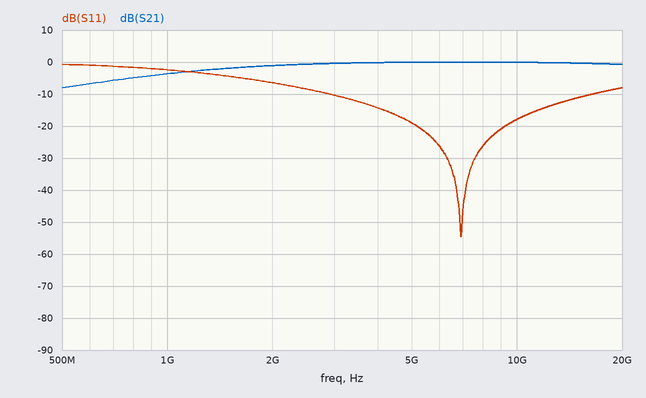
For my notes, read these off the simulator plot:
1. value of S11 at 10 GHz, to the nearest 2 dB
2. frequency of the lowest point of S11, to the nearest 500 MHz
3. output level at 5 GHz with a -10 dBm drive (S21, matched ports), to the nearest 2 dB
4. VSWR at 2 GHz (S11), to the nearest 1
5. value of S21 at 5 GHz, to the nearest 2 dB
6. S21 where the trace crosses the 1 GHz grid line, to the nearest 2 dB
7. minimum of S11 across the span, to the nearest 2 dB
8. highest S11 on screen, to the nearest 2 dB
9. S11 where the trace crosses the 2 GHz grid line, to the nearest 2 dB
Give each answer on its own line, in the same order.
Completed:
-18 dB
7.0 GHz
-10 dBm
3
0 dB
-4 dB
-54 dB
0 dB
-6 dB
